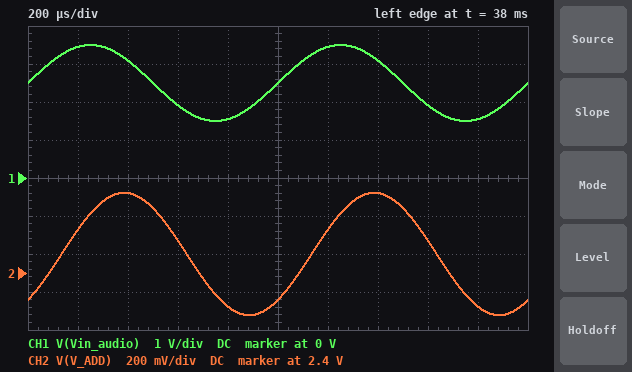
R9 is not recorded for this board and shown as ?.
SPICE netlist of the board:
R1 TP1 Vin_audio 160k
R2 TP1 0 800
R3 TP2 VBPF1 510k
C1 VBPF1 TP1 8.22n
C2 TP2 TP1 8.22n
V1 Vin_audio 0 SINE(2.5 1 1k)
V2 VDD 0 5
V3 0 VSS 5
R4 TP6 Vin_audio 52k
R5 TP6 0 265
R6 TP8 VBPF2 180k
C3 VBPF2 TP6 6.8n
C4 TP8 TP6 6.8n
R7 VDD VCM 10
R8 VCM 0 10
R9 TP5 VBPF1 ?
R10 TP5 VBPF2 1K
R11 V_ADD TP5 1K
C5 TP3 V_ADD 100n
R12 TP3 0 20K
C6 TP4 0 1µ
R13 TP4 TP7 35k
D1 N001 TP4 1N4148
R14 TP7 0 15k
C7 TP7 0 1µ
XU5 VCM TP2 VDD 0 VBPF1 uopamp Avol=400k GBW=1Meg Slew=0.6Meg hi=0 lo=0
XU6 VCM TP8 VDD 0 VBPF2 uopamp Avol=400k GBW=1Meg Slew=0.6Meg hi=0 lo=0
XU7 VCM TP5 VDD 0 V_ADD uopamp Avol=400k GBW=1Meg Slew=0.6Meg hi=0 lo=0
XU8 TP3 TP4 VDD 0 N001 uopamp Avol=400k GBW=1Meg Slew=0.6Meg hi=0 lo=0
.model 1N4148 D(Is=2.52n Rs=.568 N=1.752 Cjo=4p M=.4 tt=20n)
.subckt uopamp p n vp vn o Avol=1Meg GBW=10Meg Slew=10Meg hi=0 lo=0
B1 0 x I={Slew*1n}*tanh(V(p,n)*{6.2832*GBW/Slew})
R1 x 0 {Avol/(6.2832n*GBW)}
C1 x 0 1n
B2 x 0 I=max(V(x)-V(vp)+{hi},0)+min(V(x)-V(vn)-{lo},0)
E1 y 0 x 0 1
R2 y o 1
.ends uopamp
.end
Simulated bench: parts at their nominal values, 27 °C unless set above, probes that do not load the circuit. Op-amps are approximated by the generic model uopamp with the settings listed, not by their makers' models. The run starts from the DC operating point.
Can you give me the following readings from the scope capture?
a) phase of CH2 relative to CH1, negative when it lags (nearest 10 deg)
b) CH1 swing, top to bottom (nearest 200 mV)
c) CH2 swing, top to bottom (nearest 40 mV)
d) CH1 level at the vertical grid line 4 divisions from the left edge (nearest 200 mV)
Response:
-50 deg
2.0 V
640 mV
1.6 V
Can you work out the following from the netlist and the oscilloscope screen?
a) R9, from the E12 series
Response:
2.7 kΩ
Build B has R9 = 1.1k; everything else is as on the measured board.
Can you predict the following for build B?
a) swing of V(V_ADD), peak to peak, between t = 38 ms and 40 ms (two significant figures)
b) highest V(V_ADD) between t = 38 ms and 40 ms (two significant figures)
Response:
1.7 V
3.3 V
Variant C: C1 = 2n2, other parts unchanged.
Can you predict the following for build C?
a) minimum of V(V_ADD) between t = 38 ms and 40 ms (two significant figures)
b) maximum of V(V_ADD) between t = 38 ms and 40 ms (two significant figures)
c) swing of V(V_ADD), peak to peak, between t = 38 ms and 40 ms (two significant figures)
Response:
2.4 V
2.6 V
230 mV
